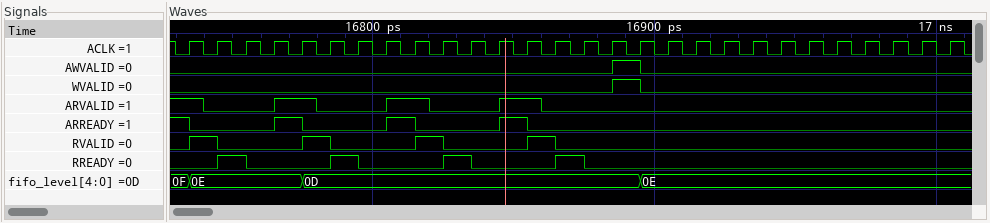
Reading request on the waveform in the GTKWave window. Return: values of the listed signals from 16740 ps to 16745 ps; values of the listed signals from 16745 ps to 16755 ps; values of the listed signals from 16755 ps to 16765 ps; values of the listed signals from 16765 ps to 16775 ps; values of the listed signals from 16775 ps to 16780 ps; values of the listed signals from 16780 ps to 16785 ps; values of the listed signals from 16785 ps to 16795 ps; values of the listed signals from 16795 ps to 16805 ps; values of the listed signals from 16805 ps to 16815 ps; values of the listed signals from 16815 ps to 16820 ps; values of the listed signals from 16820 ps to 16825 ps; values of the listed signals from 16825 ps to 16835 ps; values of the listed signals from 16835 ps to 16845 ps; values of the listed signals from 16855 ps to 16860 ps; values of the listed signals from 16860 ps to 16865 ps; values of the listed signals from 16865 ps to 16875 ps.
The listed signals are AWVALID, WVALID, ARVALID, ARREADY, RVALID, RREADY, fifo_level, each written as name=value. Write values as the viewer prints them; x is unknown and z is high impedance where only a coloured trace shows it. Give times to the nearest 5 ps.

AWVALID=0, WVALID=0, ARVALID=0, ARREADY=0, RVALID=1, RREADY=0, fifo_level=0E
AWVALID=0, WVALID=0, ARVALID=0, ARREADY=0, RVALID=0, RREADY=1, fifo_level=0E
AWVALID=0, WVALID=0, ARVALID=0, ARREADY=0, RVALID=0, RREADY=0, fifo_level=0E
AWVALID=0, WVALID=0, ARVALID=1, ARREADY=1, RVALID=0, RREADY=0, fifo_level=0E
AWVALID=0, WVALID=0, ARVALID=1, ARREADY=0, RVALID=1, RREADY=0, fifo_level=0D
AWVALID=0, WVALID=0, ARVALID=0, ARREADY=0, RVALID=1, RREADY=0, fifo_level=0D
AWVALID=0, WVALID=0, ARVALID=0, ARREADY=0, RVALID=0, RREADY=1, fifo_level=0D
AWVALID=0, WVALID=0, ARVALID=0, ARREADY=0, RVALID=0, RREADY=0, fifo_level=0D
AWVALID=0, WVALID=0, ARVALID=1, ARREADY=1, RVALID=0, RREADY=0, fifo_level=0D
AWVALID=0, WVALID=0, ARVALID=1, ARREADY=0, RVALID=1, RREADY=0, fifo_level=0D
AWVALID=0, WVALID=0, ARVALID=0, ARREADY=0, RVALID=1, RREADY=0, fifo_level=0D
AWVALID=0, WVALID=0, ARVALID=0, ARREADY=0, RVALID=0, RREADY=1, fifo_level=0D
AWVALID=0, WVALID=0, ARVALID=0, ARREADY=0, RVALID=0, RREADY=0, fifo_level=0D
AWVALID=0, WVALID=0, ARVALID=1, ARREADY=0, RVALID=1, RREADY=0, fifo_level=0D
AWVALID=0, WVALID=0, ARVALID=0, ARREADY=0, RVALID=1, RREADY=0, fifo_level=0D
AWVALID=0, WVALID=0, ARVALID=0, ARREADY=0, RVALID=0, RREADY=1, fifo_level=0D
